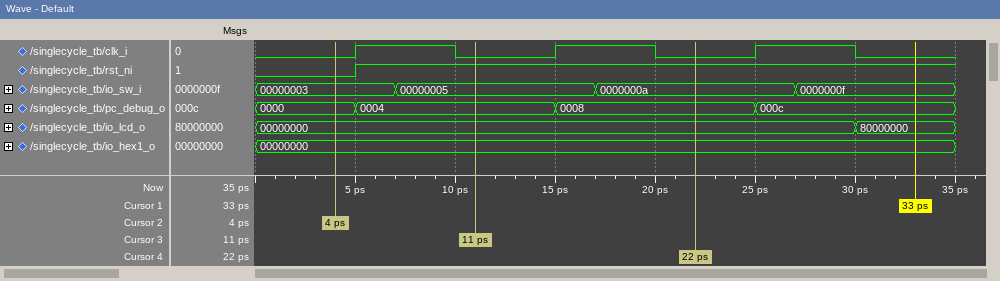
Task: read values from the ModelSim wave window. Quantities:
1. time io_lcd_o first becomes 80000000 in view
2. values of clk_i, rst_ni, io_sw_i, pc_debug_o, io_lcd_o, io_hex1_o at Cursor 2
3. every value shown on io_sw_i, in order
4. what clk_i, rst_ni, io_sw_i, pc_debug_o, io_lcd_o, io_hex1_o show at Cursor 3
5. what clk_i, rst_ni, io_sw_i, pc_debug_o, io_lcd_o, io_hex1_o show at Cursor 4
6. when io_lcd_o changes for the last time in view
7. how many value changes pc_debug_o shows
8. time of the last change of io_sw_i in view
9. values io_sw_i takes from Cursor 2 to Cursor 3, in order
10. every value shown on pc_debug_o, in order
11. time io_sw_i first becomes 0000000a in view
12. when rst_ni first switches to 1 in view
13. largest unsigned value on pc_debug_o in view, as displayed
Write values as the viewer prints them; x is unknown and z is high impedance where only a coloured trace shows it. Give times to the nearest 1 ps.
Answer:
30 ps
clk_i=0, rst_ni=0, io_sw_i=00000003, pc_debug_o=0000, io_lcd_o=00000000, io_hex1_o=00000000
00000003, 00000005, 0000000a, 0000000f
clk_i=0, rst_ni=1, io_sw_i=00000005, pc_debug_o=0004, io_lcd_o=00000000, io_hex1_o=00000000
clk_i=0, rst_ni=1, io_sw_i=0000000a, pc_debug_o=0008, io_lcd_o=00000000, io_hex1_o=00000000
30 ps
3
27 ps
00000003, 00000005
0000, 0004, 0008, 000c
17 ps
5 ps
000c
